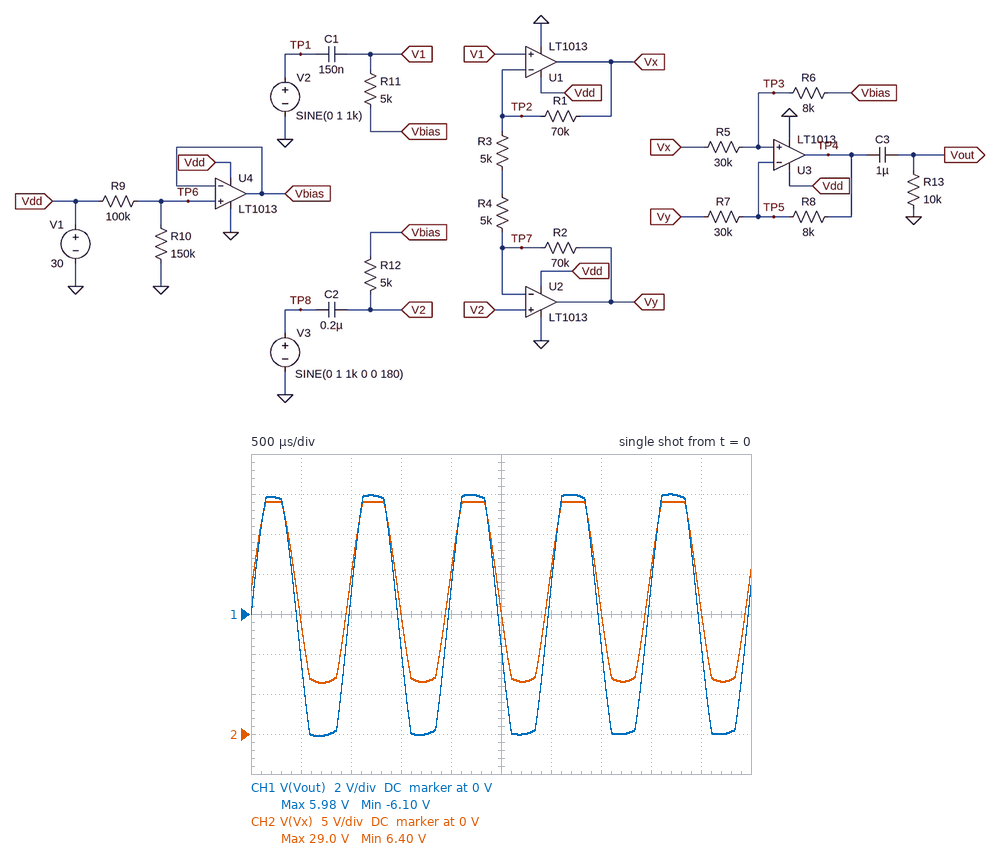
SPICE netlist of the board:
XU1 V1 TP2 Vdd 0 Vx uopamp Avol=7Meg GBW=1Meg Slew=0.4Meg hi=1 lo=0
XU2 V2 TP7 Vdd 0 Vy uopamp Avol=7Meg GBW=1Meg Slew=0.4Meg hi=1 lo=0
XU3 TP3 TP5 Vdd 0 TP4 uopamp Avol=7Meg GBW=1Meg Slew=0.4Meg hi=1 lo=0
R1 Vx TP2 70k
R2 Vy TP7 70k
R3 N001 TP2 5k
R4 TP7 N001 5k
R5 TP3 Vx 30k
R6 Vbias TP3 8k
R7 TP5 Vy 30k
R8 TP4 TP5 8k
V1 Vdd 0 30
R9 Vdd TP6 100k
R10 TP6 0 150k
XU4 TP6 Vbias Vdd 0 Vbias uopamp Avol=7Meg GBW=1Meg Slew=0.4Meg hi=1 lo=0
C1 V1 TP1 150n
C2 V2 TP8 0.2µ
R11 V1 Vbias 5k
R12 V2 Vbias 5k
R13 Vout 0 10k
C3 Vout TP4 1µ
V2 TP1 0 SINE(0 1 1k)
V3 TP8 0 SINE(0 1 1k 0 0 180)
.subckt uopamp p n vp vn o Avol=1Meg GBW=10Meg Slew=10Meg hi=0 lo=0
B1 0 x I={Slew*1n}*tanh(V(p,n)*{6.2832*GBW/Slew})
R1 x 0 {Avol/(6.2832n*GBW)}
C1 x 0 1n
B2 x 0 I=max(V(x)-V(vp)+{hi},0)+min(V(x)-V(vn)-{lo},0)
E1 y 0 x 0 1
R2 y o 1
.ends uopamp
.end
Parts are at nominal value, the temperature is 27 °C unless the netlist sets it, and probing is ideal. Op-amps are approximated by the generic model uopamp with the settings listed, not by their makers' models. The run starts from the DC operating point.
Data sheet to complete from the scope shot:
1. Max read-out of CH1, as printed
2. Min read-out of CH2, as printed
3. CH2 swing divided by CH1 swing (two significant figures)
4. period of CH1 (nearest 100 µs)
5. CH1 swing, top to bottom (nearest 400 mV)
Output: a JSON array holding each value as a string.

["5.98 V", "6.40 V", "1.9", "1.0 ms", "12.0 V"]
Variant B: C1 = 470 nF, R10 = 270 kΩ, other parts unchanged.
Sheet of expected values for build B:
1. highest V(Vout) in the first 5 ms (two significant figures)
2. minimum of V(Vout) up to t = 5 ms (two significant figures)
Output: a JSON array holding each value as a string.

["4.0 V", "-4.1 V"]
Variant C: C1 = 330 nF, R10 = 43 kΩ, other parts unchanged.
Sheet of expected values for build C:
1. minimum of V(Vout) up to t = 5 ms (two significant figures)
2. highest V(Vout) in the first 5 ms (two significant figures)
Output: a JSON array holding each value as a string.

["-5.1 V", "5.0 V"]
